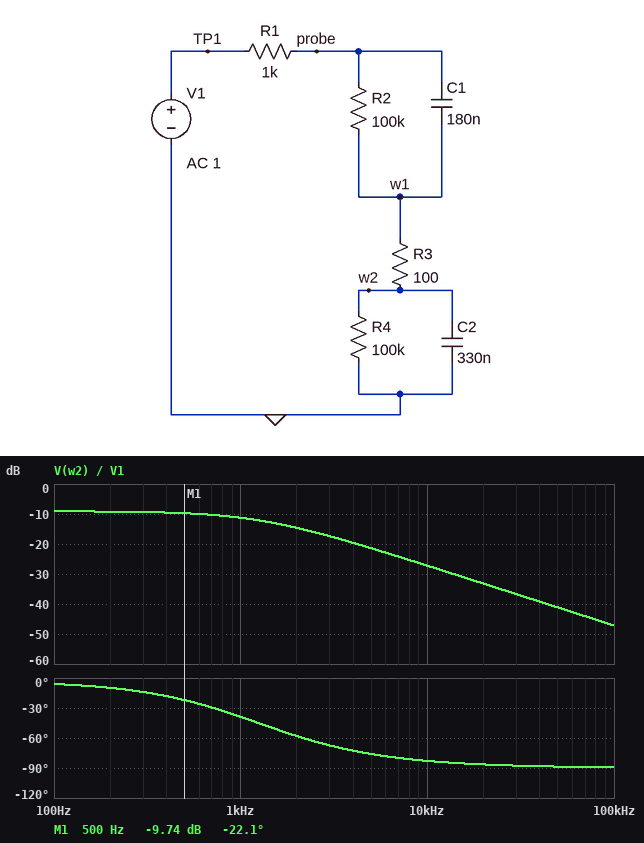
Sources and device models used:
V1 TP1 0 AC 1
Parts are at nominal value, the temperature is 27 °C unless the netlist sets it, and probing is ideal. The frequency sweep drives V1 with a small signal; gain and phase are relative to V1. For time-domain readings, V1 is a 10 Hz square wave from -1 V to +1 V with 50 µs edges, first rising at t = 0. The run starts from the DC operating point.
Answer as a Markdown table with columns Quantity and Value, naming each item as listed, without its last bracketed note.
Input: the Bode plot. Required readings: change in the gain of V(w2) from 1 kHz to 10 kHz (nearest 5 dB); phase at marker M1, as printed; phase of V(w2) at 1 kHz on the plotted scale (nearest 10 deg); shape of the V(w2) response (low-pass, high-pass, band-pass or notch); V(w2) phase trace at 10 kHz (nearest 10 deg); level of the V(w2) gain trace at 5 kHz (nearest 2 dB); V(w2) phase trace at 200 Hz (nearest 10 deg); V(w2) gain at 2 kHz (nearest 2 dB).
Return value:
| Quantity | Value |
|---|---|
| change in the gain of V(w2) from 1 kHz to 10 kHz | -15 dB |
| phase at marker M1, as printed | -22.1 deg |
| phase of V(w2) at 1 kHz on the plotted scale | -40 deg |
| shape of the V(w2) response | low-pass |
| V(w2) phase trace at 10 kHz | -80 deg |
| level of the V(w2) gain trace at 5 kHz | -22 dB |
| V(w2) phase trace at 200 Hz | -10 deg |
| V(w2) gain at 2 kHz | -14 dB |
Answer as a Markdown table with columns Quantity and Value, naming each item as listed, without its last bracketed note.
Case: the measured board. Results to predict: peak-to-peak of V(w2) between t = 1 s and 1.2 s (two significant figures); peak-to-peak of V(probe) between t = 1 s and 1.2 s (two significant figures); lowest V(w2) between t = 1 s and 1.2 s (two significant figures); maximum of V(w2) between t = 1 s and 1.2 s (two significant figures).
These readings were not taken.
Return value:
| Quantity | Value |
|---|---|
| peak-to-peak of V(w2) between t = 1 s and 1.2 s | 920 mV |
| peak-to-peak of V(probe) between t = 1 s and 1.2 s | 2.0 V |
| lowest V(w2) between t = 1 s and 1.2 s | -460 mV |
| maximum of V(w2) between t = 1 s and 1.2 s | 460 mV |
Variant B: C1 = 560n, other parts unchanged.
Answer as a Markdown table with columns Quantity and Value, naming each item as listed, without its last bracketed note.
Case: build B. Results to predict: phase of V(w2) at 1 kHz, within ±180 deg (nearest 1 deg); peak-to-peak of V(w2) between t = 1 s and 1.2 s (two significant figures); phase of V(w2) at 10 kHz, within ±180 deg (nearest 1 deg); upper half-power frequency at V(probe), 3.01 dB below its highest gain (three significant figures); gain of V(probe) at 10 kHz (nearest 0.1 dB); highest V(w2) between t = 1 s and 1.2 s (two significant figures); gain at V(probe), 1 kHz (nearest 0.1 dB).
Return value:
| Quantity | Value |
|---|---|
| phase of V(w2) at 1 kHz, within ±180 deg | -55 deg |
| peak-to-peak of V(w2) between t = 1 s and 1.2 s | 1.4 V |
| phase of V(w2) at 10 kHz, within ±180 deg | -86 deg |
| upper half-power frequency at V(probe), 3.01 dB below its highest gain | 706 Hz |
| gain of V(probe) at 10 kHz | -18.8 dB |
| highest V(w2) between t = 1 s and 1.2 s | 680 mV |
| gain at V(probe), 1 kHz | -4.8 dB |
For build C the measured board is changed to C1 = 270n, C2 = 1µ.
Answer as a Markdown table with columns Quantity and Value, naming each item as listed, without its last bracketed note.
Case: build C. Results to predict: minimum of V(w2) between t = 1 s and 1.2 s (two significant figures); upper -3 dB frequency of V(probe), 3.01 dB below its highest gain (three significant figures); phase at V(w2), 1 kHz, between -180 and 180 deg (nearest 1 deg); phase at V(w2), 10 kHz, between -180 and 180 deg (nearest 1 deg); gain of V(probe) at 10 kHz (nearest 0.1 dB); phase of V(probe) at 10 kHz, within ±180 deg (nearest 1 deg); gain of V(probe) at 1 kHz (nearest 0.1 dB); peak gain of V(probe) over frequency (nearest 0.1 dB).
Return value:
| Quantity | Value |
|---|---|
| minimum of V(w2) between t = 1 s and 1.2 s | -320 mV |
| upper -3 dB frequency of V(probe), 3.01 dB below its highest gain | 689 Hz |
| phase at V(w2), 1 kHz, between -180 and 180 deg | -56 deg |
| phase at V(w2), 10 kHz, between -180 and 180 deg | -86 deg |
| gain of V(probe) at 10 kHz | -18.9 dB |
| phase of V(probe) at 10 kHz, within ±180 deg | -33 deg |
| gain of V(probe) at 1 kHz | -4.9 dB |
| peak gain of V(probe) over frequency | 0 dB |
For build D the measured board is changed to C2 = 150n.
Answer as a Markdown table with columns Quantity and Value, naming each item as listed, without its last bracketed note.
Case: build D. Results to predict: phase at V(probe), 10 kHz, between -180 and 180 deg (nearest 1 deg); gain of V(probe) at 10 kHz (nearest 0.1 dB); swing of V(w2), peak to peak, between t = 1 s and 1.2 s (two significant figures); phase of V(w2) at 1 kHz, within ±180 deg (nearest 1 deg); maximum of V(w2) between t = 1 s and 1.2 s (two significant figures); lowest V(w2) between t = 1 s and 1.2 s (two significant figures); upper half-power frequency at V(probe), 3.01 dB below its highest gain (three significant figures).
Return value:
| Quantity | Value |
|---|---|
| phase at V(probe), 10 kHz, between -180 and 180 deg | -53 deg |
| gain of V(probe) at 10 kHz | -14.2 dB |
| swing of V(w2), peak to peak, between t = 1 s and 1.2 s | 1.2 V |
| phase of V(w2) at 1 kHz, within ±180 deg | -29 deg |
| maximum of V(w2) between t = 1 s and 1.2 s | 580 mV |
| lowest V(w2) between t = 1 s and 1.2 s | -580 mV |
| upper half-power frequency at V(probe), 3.01 dB below its highest gain | 1.79 kHz |
